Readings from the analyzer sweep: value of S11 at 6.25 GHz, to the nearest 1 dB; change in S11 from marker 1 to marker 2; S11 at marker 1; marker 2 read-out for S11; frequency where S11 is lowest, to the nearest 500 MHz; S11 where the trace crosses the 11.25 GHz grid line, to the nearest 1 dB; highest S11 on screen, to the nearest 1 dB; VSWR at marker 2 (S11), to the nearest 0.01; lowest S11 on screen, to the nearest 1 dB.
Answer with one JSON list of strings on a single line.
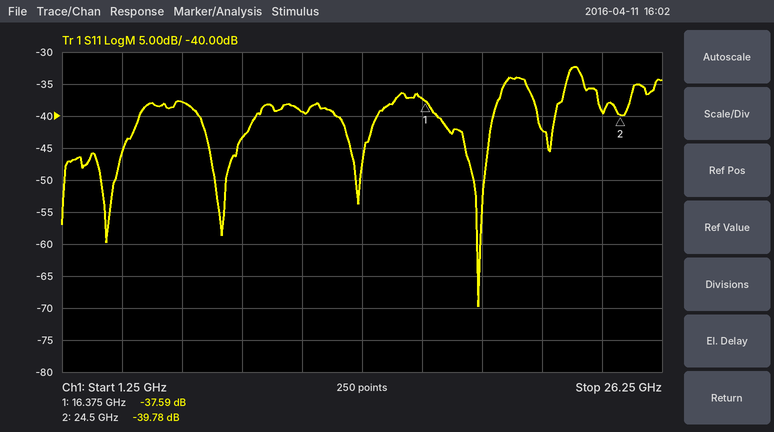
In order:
["-38 dB", "-2.19 dB", "-37.59 dB", "-39.78 dB", "18.5 GHz", "-39 dB", "-32 dB", "1.02", "-70 dB"]
